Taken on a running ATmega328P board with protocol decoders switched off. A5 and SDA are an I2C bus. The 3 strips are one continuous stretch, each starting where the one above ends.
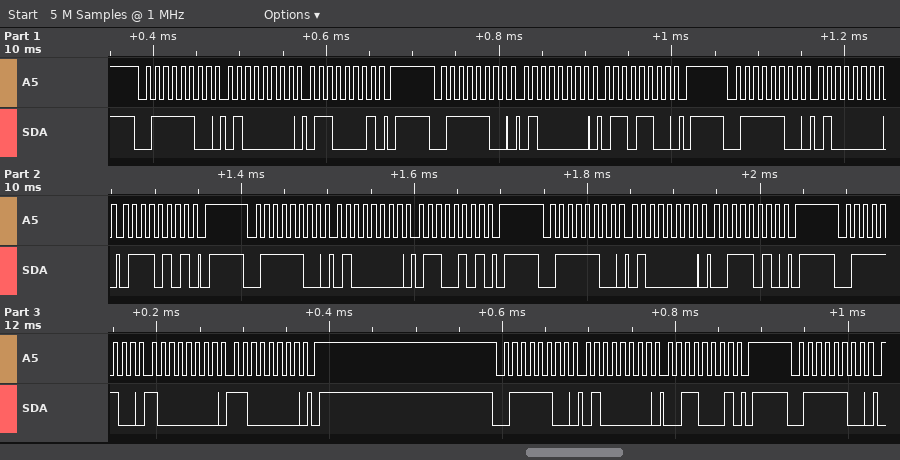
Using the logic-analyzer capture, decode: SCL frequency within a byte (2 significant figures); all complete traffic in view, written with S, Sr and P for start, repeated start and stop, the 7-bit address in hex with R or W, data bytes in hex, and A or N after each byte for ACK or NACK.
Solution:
100 kHz
S 3EW A 40 A 61 A P S 3EW A 40 A 6C A P S 3EW A 40 A 75 A P S 3EW A 40 A 65 A P S 3EW A 40 A 3A A P S 3EW A 80 A C0 A P S 3EW A 40 A 31 A P S 3EW A
